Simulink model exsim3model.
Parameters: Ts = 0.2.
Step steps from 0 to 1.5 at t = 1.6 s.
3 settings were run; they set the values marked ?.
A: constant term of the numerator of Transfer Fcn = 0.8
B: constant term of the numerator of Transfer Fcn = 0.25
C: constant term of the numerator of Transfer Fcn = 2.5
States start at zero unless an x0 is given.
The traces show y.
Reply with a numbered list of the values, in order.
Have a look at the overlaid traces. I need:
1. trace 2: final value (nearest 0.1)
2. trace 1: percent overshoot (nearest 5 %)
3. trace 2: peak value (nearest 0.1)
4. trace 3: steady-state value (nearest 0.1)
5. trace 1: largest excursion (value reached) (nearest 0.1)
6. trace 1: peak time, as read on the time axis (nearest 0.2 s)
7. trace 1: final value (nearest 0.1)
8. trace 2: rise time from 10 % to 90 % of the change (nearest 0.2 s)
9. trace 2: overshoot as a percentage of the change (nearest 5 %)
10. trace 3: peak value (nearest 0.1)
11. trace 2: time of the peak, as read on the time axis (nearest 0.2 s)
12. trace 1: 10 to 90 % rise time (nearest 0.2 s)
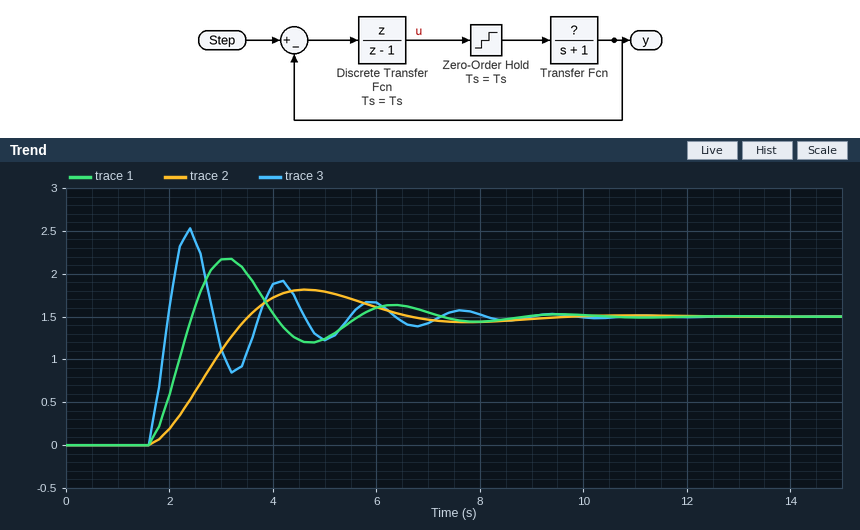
1. 1.5
2. 45 %
3. 1.8
4. 1.5
5. 2.2
6. 3.2 s
7. 1.5
8. 1.4 s
9. 20 %
10. 2.5
11. 4.6 s
12. 0.6 s
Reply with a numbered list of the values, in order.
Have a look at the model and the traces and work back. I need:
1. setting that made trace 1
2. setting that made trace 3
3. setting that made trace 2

1. A
2. C
3. B
